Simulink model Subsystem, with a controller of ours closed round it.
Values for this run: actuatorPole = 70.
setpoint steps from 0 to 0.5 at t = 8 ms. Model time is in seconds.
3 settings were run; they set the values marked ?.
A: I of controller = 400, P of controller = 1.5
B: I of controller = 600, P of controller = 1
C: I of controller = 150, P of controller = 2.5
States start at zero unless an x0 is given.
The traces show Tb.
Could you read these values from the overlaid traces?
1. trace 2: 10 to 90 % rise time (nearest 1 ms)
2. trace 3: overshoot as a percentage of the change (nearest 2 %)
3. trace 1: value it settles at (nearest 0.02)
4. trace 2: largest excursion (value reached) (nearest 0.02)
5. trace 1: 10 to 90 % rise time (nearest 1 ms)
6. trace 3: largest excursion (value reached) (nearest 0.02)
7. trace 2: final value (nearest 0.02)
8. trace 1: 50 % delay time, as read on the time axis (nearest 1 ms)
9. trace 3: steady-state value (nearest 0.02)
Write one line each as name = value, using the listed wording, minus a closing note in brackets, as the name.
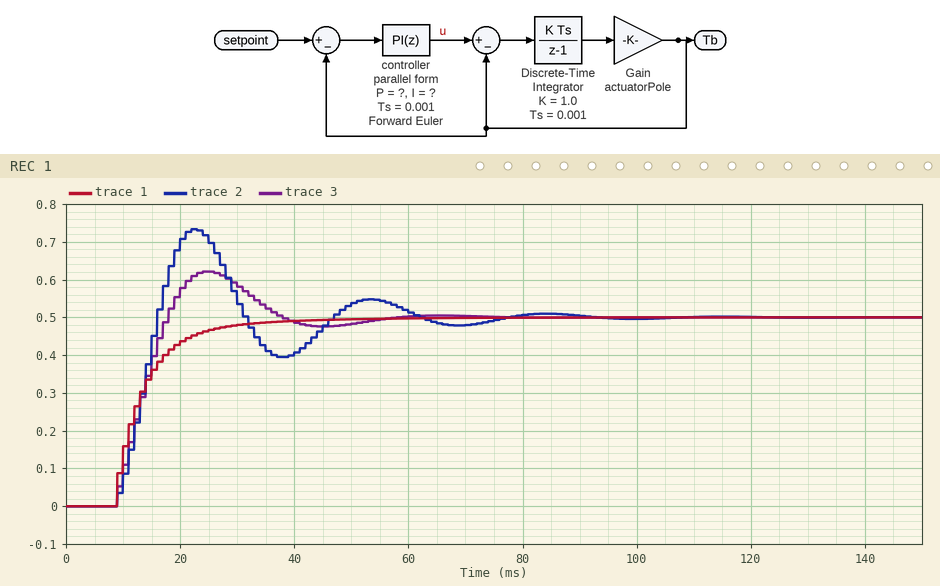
trace 2: 10 to 90 % rise time = 5 ms
trace 3: overshoot as a percentage of the change = 24 %
trace 1: value it settles at = 0.50
trace 2: largest excursion (value reached) = 0.74
trace 1: 10 to 90 % rise time = 13 ms
trace 3: largest excursion (value reached) = 0.62
trace 2: final value = 0.50
trace 1: 50 % delay time, as read on the time axis = 12 ms
trace 3: steady-state value = 0.50
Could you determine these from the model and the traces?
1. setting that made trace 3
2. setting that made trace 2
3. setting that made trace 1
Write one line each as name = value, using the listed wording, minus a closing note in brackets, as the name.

setting that made trace 3 = A
setting that made trace 2 = B
setting that made trace 1 = C
